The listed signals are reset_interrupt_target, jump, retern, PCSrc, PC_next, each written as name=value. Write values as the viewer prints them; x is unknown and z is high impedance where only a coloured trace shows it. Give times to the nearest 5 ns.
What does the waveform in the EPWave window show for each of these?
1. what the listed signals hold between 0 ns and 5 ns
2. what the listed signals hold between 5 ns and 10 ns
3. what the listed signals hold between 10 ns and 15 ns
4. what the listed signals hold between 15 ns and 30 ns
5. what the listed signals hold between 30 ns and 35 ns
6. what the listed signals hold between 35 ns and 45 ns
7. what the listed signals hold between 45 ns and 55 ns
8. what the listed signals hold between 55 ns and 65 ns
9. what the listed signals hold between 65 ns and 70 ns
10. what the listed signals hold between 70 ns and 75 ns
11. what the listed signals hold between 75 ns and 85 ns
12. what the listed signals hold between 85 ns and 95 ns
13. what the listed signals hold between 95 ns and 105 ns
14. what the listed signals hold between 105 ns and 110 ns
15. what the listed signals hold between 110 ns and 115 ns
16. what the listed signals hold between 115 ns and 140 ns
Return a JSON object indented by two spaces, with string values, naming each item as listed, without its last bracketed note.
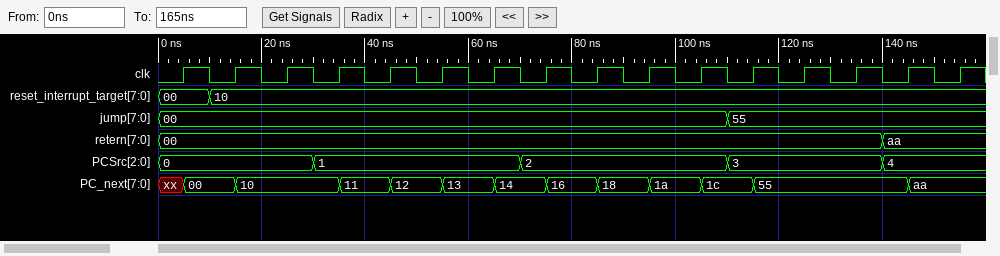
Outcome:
{
  "what the listed signals hold between 0 ns and 5 ns": "reset_interrupt_target=00, jump=00, retern=00, PCSrc=0, PC_next=xx",
  "what the listed signals hold between 5 ns and 10 ns": "reset_interrupt_target=00, jump=00, retern=00, PCSrc=0, PC_next=00",
  "what the listed signals hold between 10 ns and 15 ns": "reset_interrupt_target=10, jump=00, retern=00, PCSrc=0, PC_next=00",
  "what the listed signals hold between 15 ns and 30 ns": "reset_interrupt_target=10, jump=00, retern=00, PCSrc=0, PC_next=10",
  "what the listed signals hold between 30 ns and 35 ns": "reset_interrupt_target=10, jump=00, retern=00, PCSrc=1, PC_next=10",
  "what the listed signals hold between 35 ns and 45 ns": "reset_interrupt_target=10, jump=00, retern=00, PCSrc=1, PC_next=11",
  "what the listed signals hold between 45 ns and 55 ns": "reset_interrupt_target=10, jump=00, retern=00, PCSrc=1, PC_next=12",
  "what the listed signals hold between 55 ns and 65 ns": "reset_interrupt_target=10, jump=00, retern=00, PCSrc=1, PC_next=13",
  "what the listed signals hold between 65 ns and 70 ns": "reset_interrupt_target=10, jump=00, retern=00, PCSrc=1, PC_next=14",
  "what the listed signals hold between 70 ns and 75 ns": "reset_interrupt_target=10, jump=00, retern=00, PCSrc=2, PC_next=14",
  "what the listed signals hold between 75 ns and 85 ns": "reset_interrupt_target=10, jump=00, retern=00, PCSrc=2, PC_next=16",
  "what the listed signals hold between 85 ns and 95 ns": "reset_interrupt_target=10, jump=00, retern=00, PCSrc=2, PC_next=18",
  "what the listed signals hold between 95 ns and 105 ns": "reset_interrupt_target=10, jump=00, retern=00, PCSrc=2, PC_next=1a",
  "what the listed signals hold between 105 ns and 110 ns": "reset_interrupt_target=10, jump=00, retern=00, PCSrc=2, PC_next=1c",
  "what the listed signals hold between 110 ns and 115 ns": "reset_interrupt_target=10, jump=55, retern=00, PCSrc=3, PC_next=1c",
  "what the listed signals hold between 115 ns and 140 ns": "reset_interrupt_target=10, jump=55, retern=00, PCSrc=3, PC_next=55"
}
